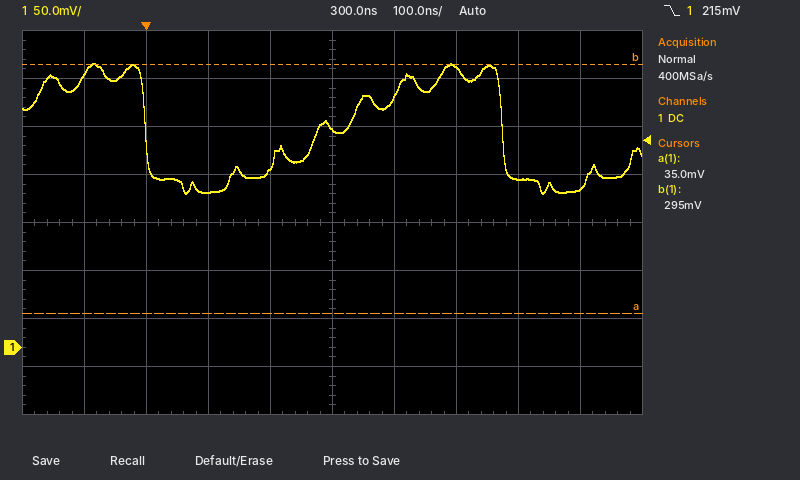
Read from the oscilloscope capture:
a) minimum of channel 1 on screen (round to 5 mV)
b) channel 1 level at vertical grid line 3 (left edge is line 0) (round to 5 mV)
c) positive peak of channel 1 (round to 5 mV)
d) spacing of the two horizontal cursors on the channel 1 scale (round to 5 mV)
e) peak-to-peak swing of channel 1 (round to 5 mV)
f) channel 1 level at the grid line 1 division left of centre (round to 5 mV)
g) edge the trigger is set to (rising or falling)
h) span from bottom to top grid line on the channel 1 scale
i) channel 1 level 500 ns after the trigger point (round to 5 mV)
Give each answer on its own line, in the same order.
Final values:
160 mV
160 mV
295 mV
260 mV
135 mV
185 mV
falling
400 mV
290 mV
